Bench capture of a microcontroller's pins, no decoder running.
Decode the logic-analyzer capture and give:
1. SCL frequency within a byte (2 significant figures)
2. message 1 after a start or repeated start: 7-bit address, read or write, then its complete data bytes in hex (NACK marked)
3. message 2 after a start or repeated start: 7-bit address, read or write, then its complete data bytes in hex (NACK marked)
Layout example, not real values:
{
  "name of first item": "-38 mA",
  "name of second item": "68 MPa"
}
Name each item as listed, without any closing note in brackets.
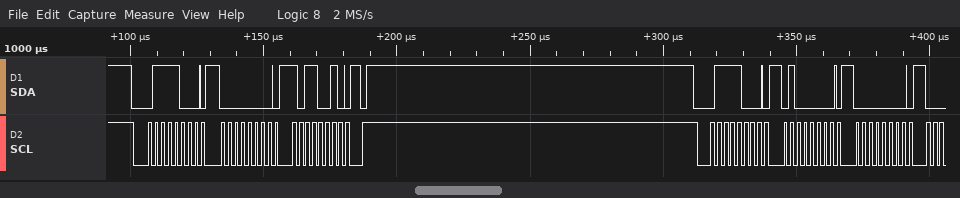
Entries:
{
  "SCL frequency within a byte": "400 kHz",
  "message 1 after a start or repeated start: 7-bit address, read or write, then its complete data bytes in hex": "0x3C write: 00 B2",
  "message 2 after a start or repeated start: 7-bit address, read or write, then its complete data bytes in hex": "0x3C write: 40 00"
}
